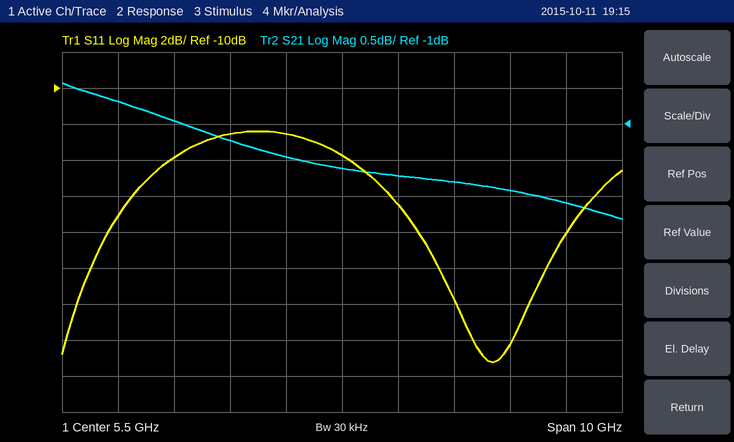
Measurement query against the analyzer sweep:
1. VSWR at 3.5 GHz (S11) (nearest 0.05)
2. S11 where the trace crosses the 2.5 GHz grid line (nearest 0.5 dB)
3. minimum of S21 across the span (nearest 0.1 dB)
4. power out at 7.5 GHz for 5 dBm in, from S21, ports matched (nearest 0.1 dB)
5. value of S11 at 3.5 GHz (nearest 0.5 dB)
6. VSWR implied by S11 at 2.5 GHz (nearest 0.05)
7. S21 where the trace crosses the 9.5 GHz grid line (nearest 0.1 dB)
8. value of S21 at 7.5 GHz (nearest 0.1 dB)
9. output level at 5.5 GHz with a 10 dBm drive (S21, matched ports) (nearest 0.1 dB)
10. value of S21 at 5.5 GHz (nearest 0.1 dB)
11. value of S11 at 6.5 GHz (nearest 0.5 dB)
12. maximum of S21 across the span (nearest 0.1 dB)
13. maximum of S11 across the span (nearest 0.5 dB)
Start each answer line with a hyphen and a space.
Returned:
- 1.60
- -14.0 dB
- -2.3 dB
- 3.2 dBm
- -12.5 dB
- 1.50
- -2.1 dB
- -1.8 dB
- 8.4 dBm
- -1.6 dB
- -16.5 dB
- -0.4 dB
- -12.5 dB
